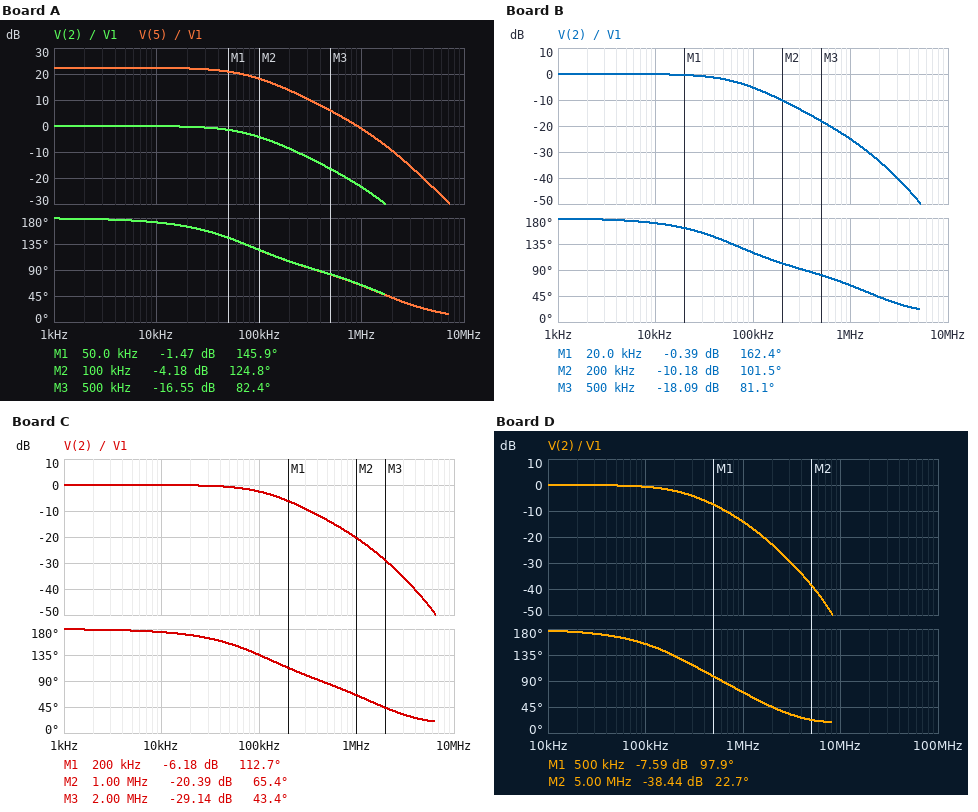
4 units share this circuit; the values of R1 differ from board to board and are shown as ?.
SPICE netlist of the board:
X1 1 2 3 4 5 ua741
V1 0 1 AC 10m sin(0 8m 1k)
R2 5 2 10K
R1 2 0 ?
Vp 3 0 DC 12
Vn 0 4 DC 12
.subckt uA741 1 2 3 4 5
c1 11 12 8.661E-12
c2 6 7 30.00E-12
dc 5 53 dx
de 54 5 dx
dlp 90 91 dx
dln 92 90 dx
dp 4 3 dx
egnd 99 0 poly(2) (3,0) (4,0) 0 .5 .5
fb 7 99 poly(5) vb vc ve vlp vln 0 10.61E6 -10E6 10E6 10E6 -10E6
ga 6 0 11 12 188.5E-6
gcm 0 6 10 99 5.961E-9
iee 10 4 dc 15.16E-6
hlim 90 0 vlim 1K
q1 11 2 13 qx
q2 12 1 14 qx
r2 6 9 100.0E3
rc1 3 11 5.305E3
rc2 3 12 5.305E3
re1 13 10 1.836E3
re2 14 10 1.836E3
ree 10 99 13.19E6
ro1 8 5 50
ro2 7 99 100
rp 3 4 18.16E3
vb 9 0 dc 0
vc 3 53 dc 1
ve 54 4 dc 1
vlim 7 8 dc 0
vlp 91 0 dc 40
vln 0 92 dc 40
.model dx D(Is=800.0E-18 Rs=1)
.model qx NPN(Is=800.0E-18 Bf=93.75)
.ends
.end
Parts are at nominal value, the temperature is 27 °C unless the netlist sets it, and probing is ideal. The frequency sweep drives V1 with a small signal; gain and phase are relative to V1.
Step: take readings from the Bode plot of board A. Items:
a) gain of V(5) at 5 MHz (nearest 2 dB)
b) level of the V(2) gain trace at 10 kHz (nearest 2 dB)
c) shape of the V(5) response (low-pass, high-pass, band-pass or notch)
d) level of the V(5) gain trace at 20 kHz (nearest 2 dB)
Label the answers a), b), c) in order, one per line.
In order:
a) -24 dB
b) 0 dB
c) low-pass
d) 22 dB
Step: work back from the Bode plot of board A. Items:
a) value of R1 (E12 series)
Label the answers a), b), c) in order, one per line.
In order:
a) 820 Ω
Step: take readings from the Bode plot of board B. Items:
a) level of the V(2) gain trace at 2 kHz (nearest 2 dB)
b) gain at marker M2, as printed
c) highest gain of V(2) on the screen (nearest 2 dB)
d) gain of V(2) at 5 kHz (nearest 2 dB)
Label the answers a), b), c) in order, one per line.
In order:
a) 0 dB
b) -10.18 dB
c) 0 dB
d) 0 dB
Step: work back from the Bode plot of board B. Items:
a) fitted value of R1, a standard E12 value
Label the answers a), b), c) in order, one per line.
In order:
a) 680 Ω
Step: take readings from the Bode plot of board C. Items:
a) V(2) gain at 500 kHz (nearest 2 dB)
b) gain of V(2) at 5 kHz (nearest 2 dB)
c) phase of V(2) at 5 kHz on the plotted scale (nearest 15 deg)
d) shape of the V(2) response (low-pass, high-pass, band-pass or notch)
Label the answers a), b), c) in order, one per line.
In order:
a) -14 dB
b) 0 dB
c) 180 deg
d) low-pass
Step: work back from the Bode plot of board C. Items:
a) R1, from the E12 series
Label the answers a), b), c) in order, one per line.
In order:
a) 1.2 kΩ
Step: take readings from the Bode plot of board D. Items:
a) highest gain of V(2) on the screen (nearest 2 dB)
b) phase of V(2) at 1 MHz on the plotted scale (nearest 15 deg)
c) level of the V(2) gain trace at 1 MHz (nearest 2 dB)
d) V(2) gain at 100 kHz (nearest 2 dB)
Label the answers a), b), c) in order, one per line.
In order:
a) 0 dB
b) 75 deg
c) -14 dB
d) 0 dB
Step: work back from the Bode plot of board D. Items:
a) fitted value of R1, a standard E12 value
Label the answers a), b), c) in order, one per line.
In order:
a) 2.7 kΩ
